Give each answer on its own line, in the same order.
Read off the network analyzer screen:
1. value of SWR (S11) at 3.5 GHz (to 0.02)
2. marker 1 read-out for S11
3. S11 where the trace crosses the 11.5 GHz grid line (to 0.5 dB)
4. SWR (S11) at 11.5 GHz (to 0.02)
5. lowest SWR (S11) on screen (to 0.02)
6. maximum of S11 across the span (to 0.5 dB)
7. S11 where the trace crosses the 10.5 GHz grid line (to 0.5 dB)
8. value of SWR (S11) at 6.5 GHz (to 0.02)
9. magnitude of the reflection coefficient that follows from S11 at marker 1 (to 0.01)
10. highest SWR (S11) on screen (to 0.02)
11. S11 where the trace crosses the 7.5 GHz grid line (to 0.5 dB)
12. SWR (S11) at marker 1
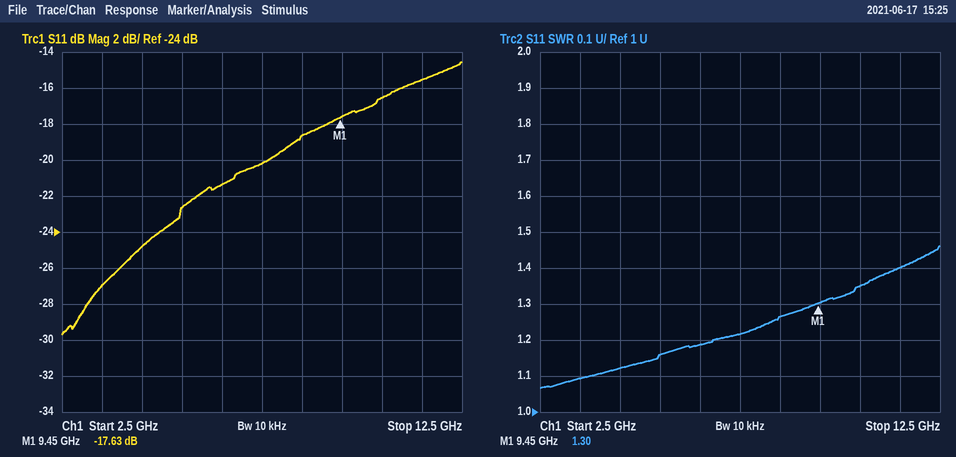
1.10
-17.63 dB
-15.5 dB
1.40
1.06
-14.5 dB
-16.5 dB
1.18
0.13
1.46
-20.0 dB
1.30
